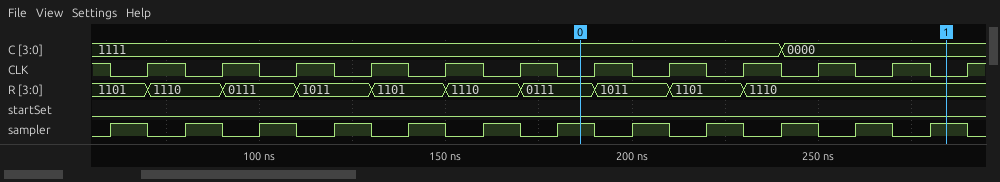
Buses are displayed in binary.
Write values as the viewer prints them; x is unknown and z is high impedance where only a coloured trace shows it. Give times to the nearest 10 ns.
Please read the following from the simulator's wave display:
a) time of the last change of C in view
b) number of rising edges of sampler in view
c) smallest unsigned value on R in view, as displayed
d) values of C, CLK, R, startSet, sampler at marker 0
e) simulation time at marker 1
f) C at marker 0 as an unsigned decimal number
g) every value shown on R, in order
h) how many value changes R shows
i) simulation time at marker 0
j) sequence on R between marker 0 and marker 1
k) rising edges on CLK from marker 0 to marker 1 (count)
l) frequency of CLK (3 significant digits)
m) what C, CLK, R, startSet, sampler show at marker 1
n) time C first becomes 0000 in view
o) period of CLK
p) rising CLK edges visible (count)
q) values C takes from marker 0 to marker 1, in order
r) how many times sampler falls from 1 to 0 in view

240 ns
12
0111
C=1111, CLK=0, R=0111, startSet=0, sampler=1
280 ns
15
1101, 1110, 0111, 1011, 1101, 1110, 0111, 1011, 1101, 1110
9
190 ns
0111, 1011, 1101, 1110
5
50.0 MHz
C=0000, CLK=0, R=1110, startSet=0, sampler=1
240 ns
20 ns
12
1111, 0000
12
